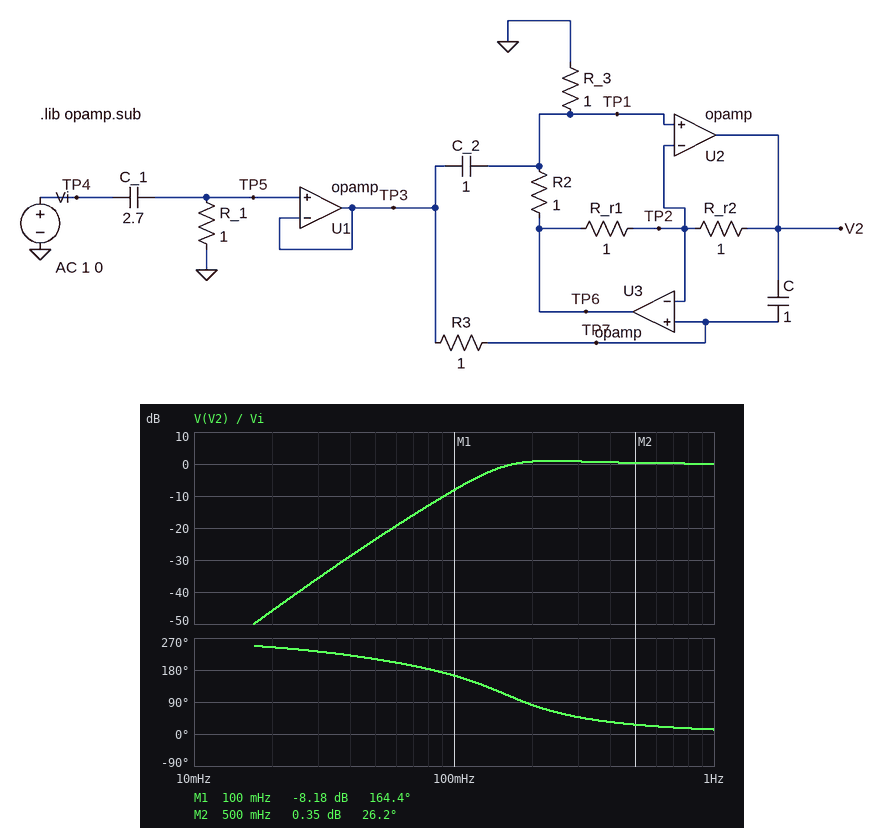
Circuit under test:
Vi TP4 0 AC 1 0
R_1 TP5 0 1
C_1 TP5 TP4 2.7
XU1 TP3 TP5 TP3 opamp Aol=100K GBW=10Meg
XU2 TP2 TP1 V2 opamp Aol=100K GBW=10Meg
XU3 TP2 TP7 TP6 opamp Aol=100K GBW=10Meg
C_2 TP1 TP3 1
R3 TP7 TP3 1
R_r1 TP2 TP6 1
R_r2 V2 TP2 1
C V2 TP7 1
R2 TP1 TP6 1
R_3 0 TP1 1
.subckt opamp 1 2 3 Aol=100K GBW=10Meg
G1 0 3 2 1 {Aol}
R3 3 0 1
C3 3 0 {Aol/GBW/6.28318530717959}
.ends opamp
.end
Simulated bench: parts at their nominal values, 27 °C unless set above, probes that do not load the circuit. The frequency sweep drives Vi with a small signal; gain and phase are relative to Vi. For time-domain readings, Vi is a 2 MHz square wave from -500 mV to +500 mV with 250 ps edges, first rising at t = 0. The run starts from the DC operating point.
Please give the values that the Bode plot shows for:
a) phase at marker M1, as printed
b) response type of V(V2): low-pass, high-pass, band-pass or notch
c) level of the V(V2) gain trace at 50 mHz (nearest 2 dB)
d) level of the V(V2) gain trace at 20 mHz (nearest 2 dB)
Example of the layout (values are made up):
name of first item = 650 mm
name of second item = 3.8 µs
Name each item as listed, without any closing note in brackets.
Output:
phase at marker M1, as printed = 164.4 deg
response type of V(V2): low-pass, high-pass, band-pass or notch = high-pass
level of the V(V2) gain trace at 50 mHz = -24 dB
level of the V(V2) gain trace at 20 mHz = -46 dB
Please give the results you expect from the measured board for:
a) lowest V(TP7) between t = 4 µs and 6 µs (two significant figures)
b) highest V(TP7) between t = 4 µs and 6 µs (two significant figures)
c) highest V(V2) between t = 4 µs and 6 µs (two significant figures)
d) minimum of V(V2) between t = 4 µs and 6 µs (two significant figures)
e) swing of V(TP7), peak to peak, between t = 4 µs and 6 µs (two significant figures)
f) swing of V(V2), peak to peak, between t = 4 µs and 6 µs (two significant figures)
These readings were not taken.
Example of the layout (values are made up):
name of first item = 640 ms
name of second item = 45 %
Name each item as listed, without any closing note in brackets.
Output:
lowest V(TP7) between t = 4 µs and 6 µs = -140 mV
highest V(TP7) between t = 4 µs and 6 µs = 1.1 V
highest V(V2) between t = 4 µs and 6 µs = 1.1 V
minimum of V(V2) between t = 4 µs and 6 µs = -140 mV
swing of V(TP7), peak to peak, between t = 4 µs and 6 µs = 1.3 V
swing of V(V2), peak to peak, between t = 4 µs and 6 µs = 1.3 V
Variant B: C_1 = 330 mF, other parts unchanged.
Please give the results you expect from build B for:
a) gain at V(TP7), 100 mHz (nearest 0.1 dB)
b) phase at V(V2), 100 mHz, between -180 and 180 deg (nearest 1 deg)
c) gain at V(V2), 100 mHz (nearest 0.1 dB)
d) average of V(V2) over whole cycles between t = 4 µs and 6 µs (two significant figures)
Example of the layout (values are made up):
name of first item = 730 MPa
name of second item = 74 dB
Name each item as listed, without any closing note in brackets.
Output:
gain at V(TP7), 100 mHz = -17.0 dB
phase at V(V2), 100 mHz, between -180 and 180 deg = -148 deg
gain at V(V2), 100 mHz = -20.7 dB
average of V(V2) over whole cycles between t = 4 µs and 6 µs = 500 mV
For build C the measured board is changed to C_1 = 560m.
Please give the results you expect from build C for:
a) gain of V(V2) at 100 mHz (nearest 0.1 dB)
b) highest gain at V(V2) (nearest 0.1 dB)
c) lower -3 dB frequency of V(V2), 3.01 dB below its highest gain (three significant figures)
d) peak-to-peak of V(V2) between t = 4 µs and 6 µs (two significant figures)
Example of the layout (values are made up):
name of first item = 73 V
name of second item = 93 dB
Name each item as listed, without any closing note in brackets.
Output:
gain of V(V2) at 100 mHz = -16.5 dB
highest gain at V(V2) = 0 dB
lower -3 dB frequency of V(V2), 3.01 dB below its highest gain = 220 mHz
peak-to-peak of V(V2) between t = 4 µs and 6 µs = 1.3 V
